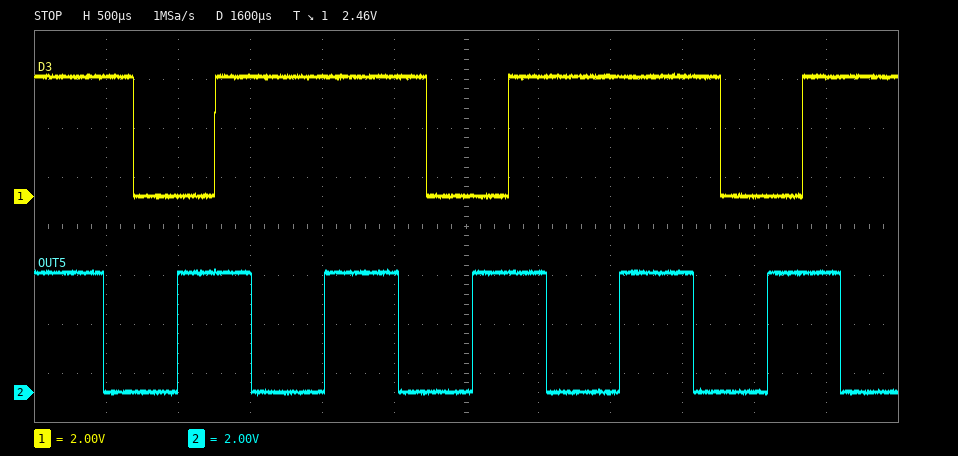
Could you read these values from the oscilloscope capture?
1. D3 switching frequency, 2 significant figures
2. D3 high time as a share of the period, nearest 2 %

490 Hz
72 %
